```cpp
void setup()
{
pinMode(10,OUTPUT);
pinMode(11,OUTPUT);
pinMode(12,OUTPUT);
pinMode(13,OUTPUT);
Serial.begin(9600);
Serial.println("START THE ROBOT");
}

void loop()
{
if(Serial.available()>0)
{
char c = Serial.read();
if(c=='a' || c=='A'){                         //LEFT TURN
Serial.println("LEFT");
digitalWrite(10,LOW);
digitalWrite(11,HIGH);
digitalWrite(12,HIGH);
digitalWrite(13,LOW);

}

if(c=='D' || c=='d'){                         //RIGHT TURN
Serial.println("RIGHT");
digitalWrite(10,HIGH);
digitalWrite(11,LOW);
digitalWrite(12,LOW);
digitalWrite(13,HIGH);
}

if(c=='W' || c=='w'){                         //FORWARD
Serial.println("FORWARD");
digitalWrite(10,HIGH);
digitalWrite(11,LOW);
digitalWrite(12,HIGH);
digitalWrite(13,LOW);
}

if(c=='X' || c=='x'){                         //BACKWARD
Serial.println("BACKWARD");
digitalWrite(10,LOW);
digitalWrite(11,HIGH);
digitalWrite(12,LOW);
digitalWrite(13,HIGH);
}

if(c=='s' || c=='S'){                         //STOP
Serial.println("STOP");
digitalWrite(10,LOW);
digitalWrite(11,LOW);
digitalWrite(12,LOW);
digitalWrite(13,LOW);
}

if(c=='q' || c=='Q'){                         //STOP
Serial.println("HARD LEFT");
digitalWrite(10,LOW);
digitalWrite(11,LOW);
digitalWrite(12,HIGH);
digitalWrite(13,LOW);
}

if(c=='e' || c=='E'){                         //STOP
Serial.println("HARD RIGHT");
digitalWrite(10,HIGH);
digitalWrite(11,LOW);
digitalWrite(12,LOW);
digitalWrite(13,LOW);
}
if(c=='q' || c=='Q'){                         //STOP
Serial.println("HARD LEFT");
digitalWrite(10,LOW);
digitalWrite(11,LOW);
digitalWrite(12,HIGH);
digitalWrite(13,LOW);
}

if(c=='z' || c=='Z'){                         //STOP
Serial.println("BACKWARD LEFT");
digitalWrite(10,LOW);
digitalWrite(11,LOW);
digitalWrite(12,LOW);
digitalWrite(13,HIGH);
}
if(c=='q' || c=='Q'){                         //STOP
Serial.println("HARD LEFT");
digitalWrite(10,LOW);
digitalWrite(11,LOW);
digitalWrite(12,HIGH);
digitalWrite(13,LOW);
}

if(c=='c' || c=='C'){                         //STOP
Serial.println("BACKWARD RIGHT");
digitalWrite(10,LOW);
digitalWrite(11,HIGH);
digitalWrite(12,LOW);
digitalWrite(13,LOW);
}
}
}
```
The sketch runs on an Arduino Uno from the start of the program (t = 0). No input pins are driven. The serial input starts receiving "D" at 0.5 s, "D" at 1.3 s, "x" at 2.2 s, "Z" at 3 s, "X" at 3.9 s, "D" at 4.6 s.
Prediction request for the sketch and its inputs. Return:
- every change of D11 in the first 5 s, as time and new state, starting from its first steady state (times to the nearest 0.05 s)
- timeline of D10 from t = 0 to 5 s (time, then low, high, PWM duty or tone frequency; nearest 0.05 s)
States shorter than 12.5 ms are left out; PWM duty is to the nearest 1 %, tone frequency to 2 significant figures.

0 s low; 2.2 s high; 3 s low; 3.9 s high; 4.6 s low
0 s low; 0.5 s high; 2.2 s low; 4.6 s high
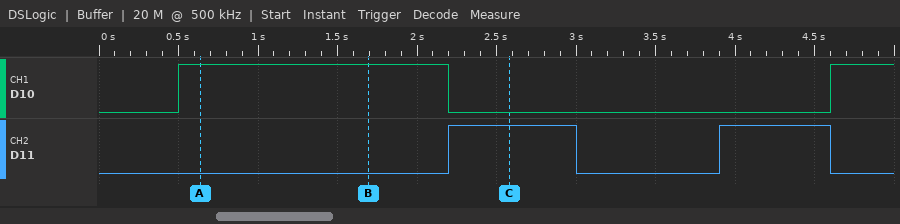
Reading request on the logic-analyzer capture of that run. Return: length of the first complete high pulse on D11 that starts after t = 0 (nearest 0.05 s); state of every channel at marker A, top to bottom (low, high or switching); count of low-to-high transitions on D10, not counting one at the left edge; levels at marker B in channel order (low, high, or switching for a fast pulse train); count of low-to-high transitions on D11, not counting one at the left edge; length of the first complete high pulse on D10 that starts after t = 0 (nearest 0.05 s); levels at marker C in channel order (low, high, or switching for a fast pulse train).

0.80 s
D10 high, D11 low
2
D10 high, D11 low
2
1.70 s
D10 low, D11 high
